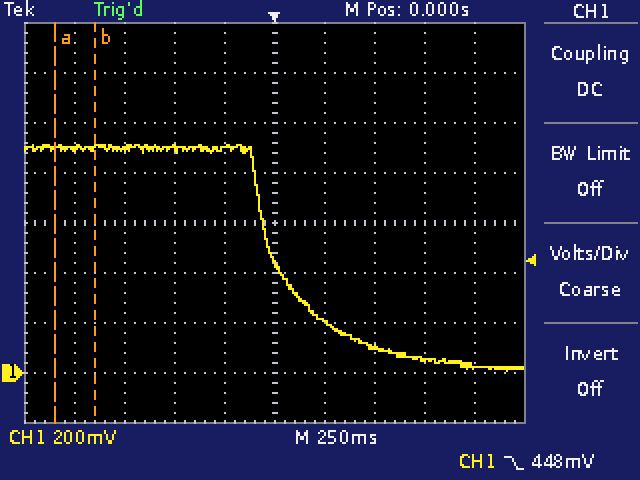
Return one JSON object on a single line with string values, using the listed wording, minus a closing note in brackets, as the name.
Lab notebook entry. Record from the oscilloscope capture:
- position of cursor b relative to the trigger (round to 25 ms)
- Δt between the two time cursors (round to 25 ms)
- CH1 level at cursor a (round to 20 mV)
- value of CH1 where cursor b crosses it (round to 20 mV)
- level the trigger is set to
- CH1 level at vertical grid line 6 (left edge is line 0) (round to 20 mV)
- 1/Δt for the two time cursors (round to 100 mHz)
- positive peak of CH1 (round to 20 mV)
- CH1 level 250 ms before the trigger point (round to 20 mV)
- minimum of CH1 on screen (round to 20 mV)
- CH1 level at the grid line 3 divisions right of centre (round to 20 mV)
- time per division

{"position of cursor b relative to the trigger": "-900 ms", "Δt between the two time cursors": "200 ms", "CH1 level at cursor a": "900 mV", "value of CH1 where cursor b crosses it": "900 mV", "level the trigger is set to": "448 mV", "CH1 level at vertical grid line 6 (left edge is line 0)": "200 mV", "1/Δt for the two time cursors": "5.0 Hz", "positive peak of CH1": "920 mV", "CH1 level 250 ms before the trigger point": "900 mV", "minimum of CH1 on screen": "0 mV", "CH1 level at the grid line 3 divisions right of centre": "60 mV", "time per division": "250 ms"}
